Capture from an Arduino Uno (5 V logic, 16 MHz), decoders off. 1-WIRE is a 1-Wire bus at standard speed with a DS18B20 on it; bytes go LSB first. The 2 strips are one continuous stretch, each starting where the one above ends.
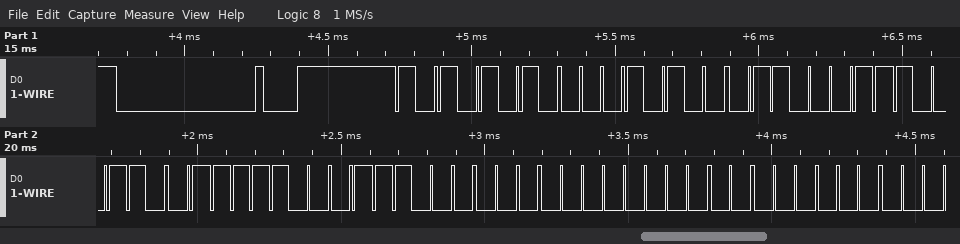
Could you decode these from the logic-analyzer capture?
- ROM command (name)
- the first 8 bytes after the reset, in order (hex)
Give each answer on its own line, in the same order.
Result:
Match ROM
55 28 C6 99 8F 03 00 00
